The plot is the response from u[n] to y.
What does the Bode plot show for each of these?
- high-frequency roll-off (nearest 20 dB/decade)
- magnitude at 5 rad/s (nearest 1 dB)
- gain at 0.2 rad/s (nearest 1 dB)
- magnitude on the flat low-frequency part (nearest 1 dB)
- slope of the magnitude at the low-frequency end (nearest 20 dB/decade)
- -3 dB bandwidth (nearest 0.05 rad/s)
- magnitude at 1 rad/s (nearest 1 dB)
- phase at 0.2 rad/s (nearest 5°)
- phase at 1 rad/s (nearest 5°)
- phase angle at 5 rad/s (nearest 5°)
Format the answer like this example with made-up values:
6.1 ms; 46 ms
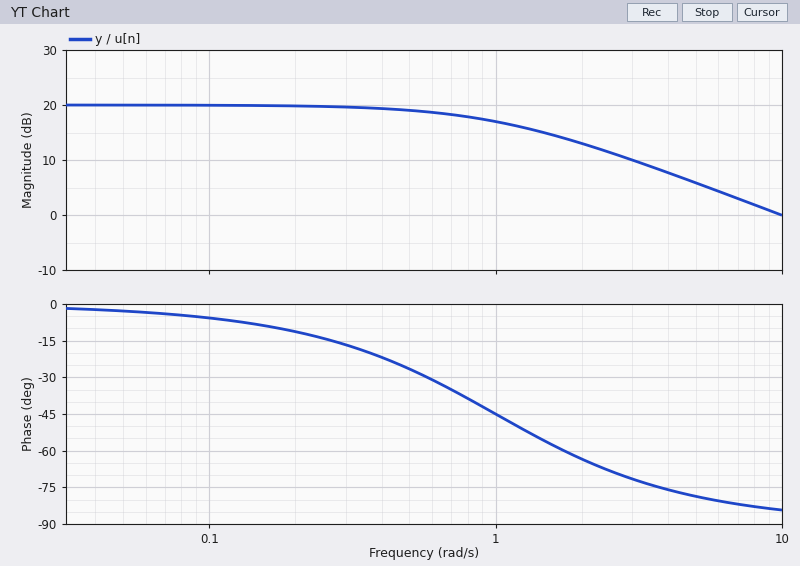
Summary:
-20 dB/decade; 6 dB; 20 dB; 20 dB; 0 dB/decade; 1.00 rad/s; 17 dB; -10°; -45°; -80°
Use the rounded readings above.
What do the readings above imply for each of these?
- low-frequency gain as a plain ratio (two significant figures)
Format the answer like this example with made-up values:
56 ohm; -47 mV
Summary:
10
